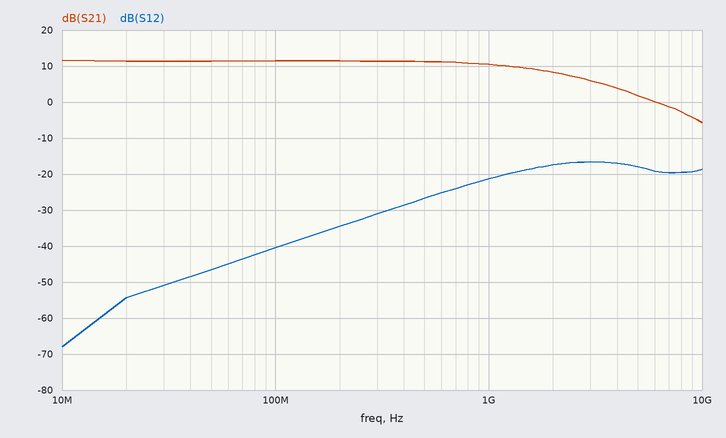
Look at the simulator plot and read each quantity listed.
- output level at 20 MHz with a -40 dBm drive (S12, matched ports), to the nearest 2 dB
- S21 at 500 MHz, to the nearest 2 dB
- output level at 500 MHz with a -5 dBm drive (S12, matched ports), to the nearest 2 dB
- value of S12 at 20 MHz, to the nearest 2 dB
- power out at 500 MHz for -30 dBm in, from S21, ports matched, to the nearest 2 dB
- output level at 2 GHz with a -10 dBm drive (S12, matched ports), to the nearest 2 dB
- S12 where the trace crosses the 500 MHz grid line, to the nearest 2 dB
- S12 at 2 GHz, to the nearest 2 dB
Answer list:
-94 dBm
12 dB
-32 dBm
-54 dB
-18 dBm
-28 dBm
-26 dB
-18 dB
